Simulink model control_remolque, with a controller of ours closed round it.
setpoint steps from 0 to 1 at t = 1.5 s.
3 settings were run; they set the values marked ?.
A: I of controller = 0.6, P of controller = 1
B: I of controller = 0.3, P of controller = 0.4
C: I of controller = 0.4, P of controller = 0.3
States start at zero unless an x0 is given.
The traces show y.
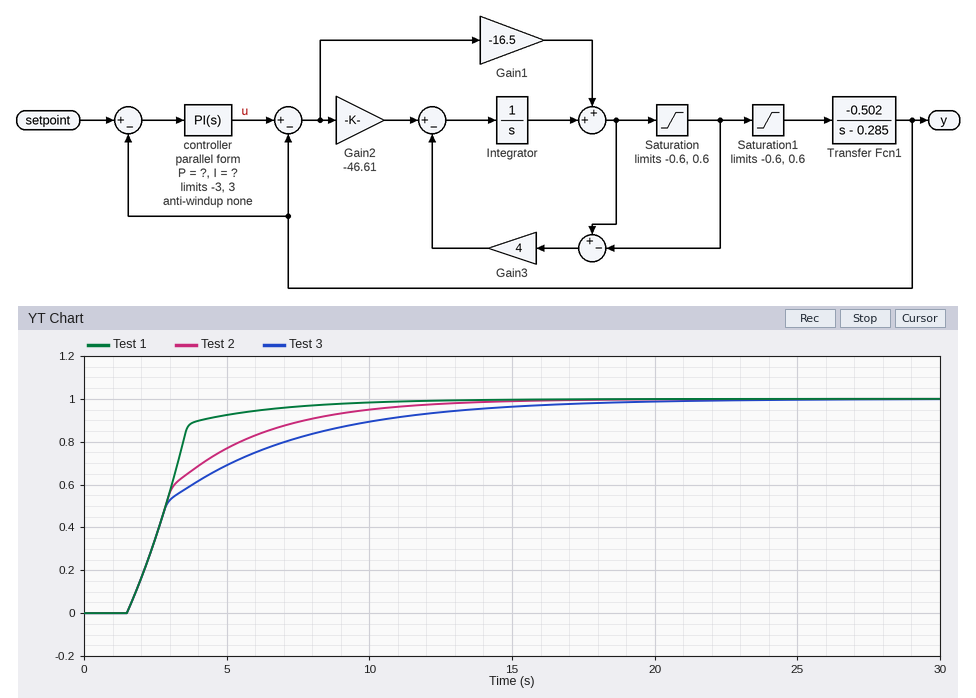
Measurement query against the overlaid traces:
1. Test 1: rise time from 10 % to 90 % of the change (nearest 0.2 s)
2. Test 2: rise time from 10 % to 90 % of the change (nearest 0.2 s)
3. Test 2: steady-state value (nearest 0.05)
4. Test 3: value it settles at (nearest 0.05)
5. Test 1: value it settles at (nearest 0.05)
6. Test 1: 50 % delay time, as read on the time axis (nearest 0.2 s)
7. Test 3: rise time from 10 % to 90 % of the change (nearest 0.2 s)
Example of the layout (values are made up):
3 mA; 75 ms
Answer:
2.2 s; 6.0 s; 1.00; 1.00; 1.00; 2.8 s; 8.4 s
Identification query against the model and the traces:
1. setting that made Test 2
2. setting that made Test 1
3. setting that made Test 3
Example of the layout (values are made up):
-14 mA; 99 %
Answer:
C; A; B
